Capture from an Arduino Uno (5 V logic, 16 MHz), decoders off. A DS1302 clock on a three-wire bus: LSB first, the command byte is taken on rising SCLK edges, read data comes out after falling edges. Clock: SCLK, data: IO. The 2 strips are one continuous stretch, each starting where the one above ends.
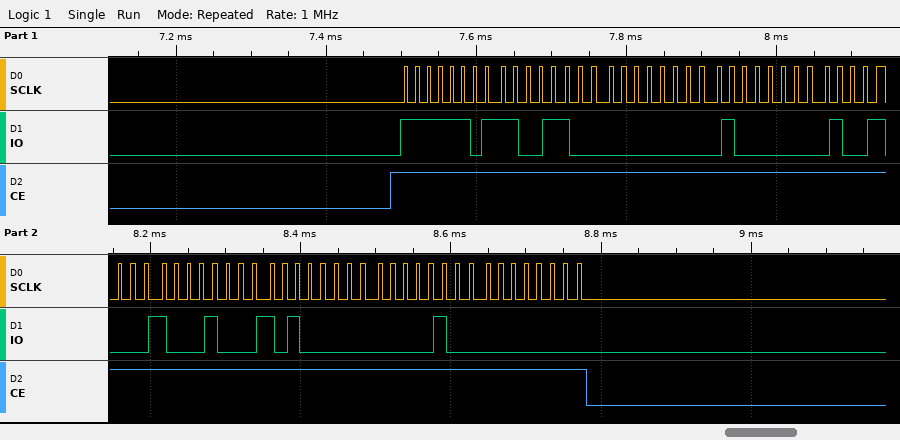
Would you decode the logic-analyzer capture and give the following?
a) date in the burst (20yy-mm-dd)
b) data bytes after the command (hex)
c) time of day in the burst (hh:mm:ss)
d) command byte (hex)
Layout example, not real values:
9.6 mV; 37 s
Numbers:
2020-11-12; 33 00 02 12 11 05 20 00; 02:00:33; 0xBF
